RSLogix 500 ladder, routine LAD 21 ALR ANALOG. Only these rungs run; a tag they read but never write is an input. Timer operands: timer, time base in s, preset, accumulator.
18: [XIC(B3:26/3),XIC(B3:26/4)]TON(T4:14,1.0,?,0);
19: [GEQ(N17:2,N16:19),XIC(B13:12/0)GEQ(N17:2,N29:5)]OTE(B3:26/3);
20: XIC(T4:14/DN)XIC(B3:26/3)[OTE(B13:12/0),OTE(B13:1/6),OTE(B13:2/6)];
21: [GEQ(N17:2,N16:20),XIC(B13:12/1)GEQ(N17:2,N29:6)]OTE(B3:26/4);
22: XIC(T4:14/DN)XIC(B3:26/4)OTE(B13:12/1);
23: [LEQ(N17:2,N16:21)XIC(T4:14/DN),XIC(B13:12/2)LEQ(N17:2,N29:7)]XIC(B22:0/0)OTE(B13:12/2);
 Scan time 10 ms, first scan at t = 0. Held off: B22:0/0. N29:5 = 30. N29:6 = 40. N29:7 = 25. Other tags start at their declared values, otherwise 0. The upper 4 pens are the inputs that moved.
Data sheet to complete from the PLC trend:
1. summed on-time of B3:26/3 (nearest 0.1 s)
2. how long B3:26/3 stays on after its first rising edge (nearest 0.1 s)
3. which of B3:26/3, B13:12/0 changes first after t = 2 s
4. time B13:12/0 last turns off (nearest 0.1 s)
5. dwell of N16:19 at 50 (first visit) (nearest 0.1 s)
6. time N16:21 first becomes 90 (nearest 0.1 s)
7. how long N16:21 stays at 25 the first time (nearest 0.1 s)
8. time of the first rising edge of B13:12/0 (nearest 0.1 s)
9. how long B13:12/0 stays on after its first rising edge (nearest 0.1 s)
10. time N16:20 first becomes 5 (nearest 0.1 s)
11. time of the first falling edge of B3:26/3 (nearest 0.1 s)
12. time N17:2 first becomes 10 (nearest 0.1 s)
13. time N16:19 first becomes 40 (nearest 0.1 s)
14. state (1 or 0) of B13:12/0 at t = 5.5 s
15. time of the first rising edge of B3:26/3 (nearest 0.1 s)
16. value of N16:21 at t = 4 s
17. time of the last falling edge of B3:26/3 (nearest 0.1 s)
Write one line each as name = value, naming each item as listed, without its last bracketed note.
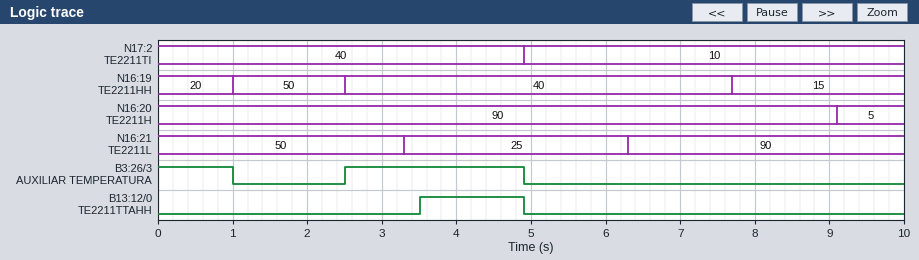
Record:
summed on-time of B3:26/3 = 3.4 s
how long B3:26/3 stays on after its first rising edge = 2.4 s
which of B3:26/3, B13:12/0 changes first after t = 2 s = B3:26/3
time B13:12/0 last turns off = 4.9 s
dwell of N16:19 at 50 (first visit) = 1.5 s
time N16:21 first becomes 90 = 6.3 s
how long N16:21 stays at 25 the first time = 3.0 s
time of the first rising edge of B13:12/0 = 3.5 s
how long B13:12/0 stays on after its first rising edge = 1.4 s
time N16:20 first becomes 5 = 9.1 s
time of the first falling edge of B3:26/3 = 1.0 s
time N17:2 first becomes 10 = 4.9 s
time N16:19 first becomes 40 = 2.5 s
state (1 or 0) of B13:12/0 at t = 5.5 s = 0
time of the first rising edge of B3:26/3 = 2.5 s
value of N16:21 at t = 4 s = 25
time of the last falling edge of B3:26/3 = 4.9 s
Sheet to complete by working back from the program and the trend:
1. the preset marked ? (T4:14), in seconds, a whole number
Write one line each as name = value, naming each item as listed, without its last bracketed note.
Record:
the preset marked ? (T4:14), in seconds, a whole number = 1 s
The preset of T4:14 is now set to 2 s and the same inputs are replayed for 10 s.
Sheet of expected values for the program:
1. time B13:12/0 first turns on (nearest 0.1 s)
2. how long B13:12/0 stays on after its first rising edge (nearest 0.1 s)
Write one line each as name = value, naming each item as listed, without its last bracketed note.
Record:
time B13:12/0 first turns on = 4.5 s
how long B13:12/0 stays on after its first rising edge = 0.4 s
